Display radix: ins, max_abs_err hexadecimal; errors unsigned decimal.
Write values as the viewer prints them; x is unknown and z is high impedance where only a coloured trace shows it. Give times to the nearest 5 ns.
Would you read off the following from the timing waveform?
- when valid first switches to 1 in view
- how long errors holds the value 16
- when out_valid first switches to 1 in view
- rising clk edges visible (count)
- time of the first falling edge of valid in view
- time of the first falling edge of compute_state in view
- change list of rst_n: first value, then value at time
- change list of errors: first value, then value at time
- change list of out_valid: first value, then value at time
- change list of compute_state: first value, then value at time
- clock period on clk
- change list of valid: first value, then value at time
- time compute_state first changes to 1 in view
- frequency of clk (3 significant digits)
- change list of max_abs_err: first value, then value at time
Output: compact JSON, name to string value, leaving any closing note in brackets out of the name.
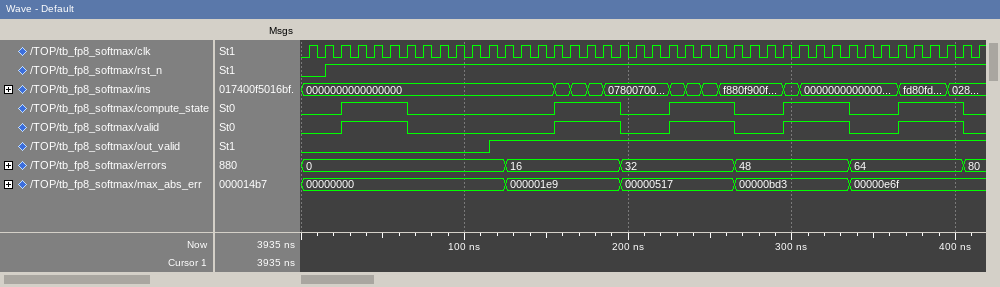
{"when valid first switches to 1 in view": "25 ns", "how long errors holds the value 16": "70 ns", "when out_valid first switches to 1 in view": "115 ns", "rising clk edges visible": "42", "time of the first falling edge of valid in view": "65 ns", "time of the first falling edge of compute_state in view": "65 ns", "change list of rst_n: first value, then value at time": "0, 1 at 15 ns", "change list of errors: first value, then value at time": "0, 16 at 125 ns, 32 at 195 ns, 48 at 265 ns, 64 at 335 ns, 80 at 405 ns", "change list of out_valid: first value, then value at time": "0, 1 at 115 ns", "change list of compute_state: first value, then value at time": "0, 1 at 25 ns, 0 at 65 ns, 1 at 155 ns, 0 at 195 ns, 1 at 225 ns, 0 at 265 ns, 1 at 295 ns, 0 at 335 ns, 1 at 365 ns, 0 at 405 ns", "clock period on clk": "10 ns", "change list of valid: first value, then value at time": "0, 1 at 25 ns, 0 at 65 ns, 1 at 155 ns, 0 at 195 ns, 1 at 225 ns, 0 at 265 ns, 1 at 295 ns, 0 at 335 ns, 1 at 365 ns, 0 at 405 ns", "time compute_state first changes to 1 in view": "25 ns", "frequency of clk": "100 MHz", "change list of max_abs_err: first value, then value at time": "00000000, 000001e9 at 125 ns, 00000517 at 195 ns, 00000bd3 at 265 ns, 00000e6f at 335 ns"}
